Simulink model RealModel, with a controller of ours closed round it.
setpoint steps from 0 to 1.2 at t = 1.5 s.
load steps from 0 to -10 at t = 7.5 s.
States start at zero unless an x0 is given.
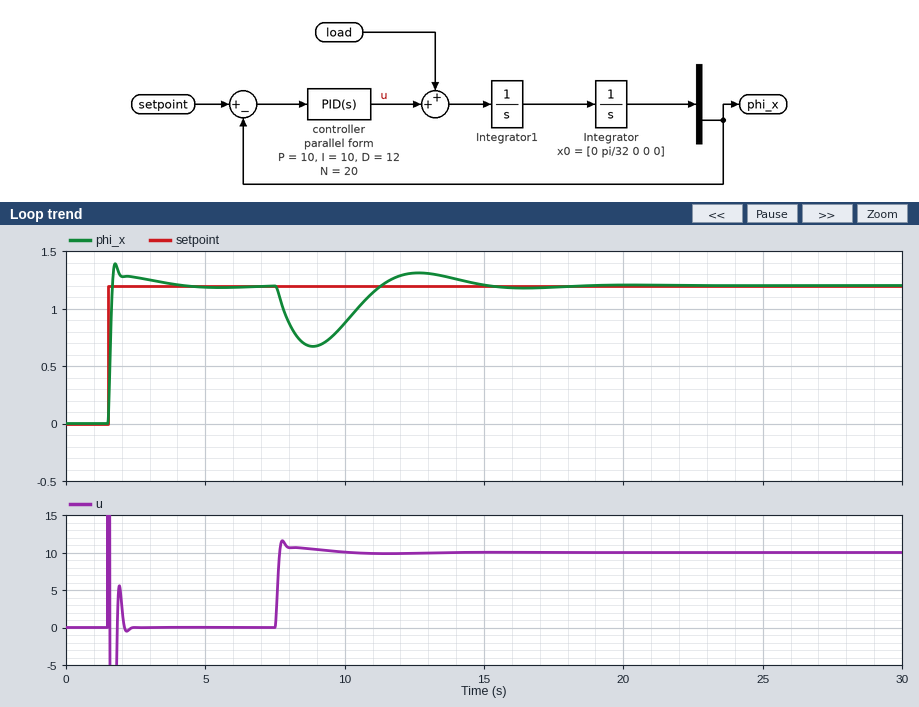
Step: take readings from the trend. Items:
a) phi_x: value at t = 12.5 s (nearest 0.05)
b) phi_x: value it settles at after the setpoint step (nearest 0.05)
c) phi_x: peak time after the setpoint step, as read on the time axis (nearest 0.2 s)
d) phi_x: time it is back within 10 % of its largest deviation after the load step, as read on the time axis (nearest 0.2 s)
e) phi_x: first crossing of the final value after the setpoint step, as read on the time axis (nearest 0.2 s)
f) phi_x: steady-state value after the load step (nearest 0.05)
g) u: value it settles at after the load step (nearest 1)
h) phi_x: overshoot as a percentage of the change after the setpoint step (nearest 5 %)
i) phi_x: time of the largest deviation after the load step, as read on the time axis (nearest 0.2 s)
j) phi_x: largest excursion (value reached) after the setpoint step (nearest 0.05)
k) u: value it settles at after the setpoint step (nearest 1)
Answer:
1.30
1.20
1.8 s
14.0 s
1.6 s
1.20
10
15 %
8.8 s
1.40
0
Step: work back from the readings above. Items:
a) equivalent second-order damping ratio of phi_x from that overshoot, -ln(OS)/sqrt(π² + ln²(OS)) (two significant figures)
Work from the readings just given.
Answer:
0.52
